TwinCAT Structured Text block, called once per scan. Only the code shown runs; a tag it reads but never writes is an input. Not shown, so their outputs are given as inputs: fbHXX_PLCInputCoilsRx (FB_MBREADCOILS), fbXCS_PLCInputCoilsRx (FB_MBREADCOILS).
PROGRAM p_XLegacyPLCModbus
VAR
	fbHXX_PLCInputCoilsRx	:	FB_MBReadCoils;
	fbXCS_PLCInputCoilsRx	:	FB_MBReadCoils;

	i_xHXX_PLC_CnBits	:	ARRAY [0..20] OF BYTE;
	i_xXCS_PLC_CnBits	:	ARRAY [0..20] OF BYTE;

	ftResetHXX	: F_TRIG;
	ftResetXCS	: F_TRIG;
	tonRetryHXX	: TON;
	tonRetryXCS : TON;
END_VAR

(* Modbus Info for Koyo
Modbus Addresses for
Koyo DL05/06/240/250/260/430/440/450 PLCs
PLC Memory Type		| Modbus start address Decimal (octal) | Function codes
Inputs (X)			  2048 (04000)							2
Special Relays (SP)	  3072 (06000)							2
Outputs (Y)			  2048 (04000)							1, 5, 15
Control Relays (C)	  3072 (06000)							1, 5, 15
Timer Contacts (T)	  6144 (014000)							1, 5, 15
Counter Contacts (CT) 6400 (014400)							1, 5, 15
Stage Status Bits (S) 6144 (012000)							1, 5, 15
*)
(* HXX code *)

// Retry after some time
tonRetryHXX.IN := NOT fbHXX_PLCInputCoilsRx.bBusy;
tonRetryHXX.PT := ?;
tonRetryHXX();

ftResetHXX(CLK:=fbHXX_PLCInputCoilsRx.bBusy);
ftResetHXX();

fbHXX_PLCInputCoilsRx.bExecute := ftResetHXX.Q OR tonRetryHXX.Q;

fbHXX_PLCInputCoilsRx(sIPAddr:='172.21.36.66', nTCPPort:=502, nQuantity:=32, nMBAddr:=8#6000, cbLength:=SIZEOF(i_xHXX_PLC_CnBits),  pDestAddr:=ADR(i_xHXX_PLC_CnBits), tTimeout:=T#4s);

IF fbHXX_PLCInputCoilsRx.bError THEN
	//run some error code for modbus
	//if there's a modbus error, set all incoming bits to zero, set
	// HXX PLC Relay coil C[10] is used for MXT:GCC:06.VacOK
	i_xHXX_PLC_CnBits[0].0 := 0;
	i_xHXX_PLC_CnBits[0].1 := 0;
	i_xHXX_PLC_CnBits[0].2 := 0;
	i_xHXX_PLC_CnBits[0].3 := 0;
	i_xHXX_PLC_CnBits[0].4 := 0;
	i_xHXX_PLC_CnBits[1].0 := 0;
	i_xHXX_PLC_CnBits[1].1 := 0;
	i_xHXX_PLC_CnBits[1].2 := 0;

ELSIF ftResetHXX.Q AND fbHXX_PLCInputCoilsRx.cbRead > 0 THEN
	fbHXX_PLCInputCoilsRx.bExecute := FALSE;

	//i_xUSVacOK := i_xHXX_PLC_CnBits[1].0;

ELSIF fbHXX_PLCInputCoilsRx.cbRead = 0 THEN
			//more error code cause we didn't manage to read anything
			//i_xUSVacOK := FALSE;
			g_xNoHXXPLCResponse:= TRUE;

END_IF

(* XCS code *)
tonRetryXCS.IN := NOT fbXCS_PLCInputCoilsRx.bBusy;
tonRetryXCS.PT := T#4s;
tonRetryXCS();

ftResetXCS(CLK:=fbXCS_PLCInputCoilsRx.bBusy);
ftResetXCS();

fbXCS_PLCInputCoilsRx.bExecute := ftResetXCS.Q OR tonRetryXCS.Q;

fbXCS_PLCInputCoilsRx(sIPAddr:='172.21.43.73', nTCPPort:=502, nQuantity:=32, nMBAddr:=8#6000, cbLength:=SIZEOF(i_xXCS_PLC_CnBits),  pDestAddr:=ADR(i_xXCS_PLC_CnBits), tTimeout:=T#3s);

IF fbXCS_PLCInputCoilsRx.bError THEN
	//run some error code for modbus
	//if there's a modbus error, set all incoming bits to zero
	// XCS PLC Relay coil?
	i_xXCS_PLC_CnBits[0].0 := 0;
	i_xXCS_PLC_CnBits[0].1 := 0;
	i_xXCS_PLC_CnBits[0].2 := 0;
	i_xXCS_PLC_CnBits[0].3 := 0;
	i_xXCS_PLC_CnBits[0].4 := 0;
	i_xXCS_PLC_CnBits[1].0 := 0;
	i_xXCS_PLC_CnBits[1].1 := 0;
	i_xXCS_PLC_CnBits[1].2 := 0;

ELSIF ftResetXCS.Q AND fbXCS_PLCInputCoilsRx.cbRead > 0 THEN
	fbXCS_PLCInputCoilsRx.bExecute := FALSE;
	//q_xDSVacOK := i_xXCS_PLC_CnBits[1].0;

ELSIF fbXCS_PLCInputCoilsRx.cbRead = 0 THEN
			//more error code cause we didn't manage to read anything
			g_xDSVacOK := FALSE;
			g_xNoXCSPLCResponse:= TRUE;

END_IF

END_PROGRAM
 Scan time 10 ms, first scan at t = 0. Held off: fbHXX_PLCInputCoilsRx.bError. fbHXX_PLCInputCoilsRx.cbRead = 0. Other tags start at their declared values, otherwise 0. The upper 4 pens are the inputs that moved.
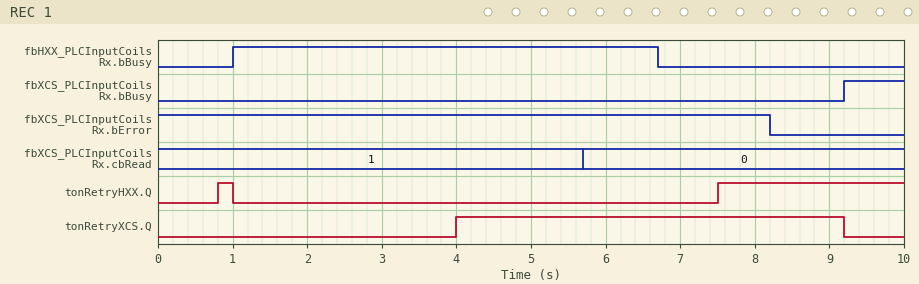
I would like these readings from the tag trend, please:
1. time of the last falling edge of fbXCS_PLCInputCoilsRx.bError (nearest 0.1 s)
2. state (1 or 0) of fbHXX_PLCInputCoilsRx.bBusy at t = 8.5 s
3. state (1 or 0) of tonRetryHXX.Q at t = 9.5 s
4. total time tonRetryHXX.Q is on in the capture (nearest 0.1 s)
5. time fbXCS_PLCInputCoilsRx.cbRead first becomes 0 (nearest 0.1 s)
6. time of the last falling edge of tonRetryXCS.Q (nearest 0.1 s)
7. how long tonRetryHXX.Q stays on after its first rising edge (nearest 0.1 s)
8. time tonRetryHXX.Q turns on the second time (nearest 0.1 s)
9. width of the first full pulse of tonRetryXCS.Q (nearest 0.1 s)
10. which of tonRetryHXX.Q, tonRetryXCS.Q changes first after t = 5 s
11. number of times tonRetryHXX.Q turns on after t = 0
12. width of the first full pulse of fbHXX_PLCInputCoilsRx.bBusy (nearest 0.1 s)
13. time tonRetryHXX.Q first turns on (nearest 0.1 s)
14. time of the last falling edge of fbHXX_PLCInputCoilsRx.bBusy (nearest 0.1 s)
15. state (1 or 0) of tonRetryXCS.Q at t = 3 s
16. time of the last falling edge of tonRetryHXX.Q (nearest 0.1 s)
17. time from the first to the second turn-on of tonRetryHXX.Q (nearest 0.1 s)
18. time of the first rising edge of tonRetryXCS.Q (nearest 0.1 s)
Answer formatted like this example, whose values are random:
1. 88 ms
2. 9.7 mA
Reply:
1. 8.2 s
2. 0
3. 1
4. 2.7 s
5. 5.7 s
6. 9.2 s
7. 0.2 s
8. 7.5 s
9. 5.2 s
10. tonRetryHXX.Q
11. 2
12. 5.7 s
13. 0.8 s
14. 6.7 s
15. 0
16. 1.0 s
17. 6.7 s
18. 4.0 s
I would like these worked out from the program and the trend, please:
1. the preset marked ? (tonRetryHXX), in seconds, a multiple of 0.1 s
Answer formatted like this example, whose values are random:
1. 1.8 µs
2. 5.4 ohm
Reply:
1. 0.8 s
